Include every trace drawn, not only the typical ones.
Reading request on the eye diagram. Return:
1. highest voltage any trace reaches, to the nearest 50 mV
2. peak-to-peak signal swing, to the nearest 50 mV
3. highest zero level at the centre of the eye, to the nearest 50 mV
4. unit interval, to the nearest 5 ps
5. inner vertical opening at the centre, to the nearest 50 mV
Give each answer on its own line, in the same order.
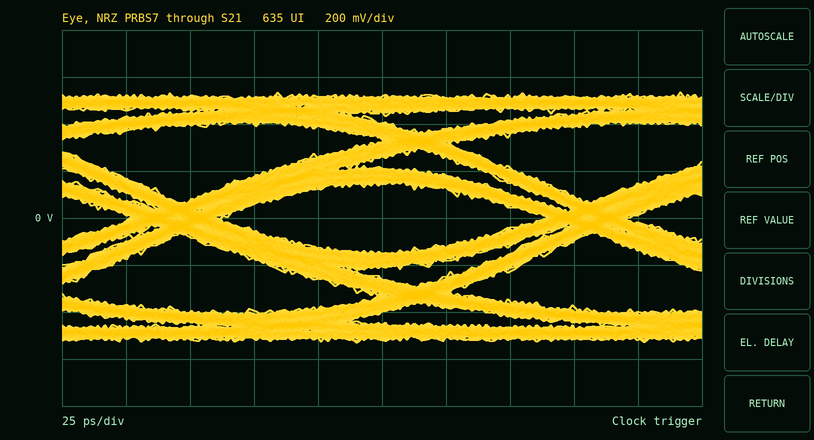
550 mV
1.05 V
-150 mV
160 ps
300 mV
